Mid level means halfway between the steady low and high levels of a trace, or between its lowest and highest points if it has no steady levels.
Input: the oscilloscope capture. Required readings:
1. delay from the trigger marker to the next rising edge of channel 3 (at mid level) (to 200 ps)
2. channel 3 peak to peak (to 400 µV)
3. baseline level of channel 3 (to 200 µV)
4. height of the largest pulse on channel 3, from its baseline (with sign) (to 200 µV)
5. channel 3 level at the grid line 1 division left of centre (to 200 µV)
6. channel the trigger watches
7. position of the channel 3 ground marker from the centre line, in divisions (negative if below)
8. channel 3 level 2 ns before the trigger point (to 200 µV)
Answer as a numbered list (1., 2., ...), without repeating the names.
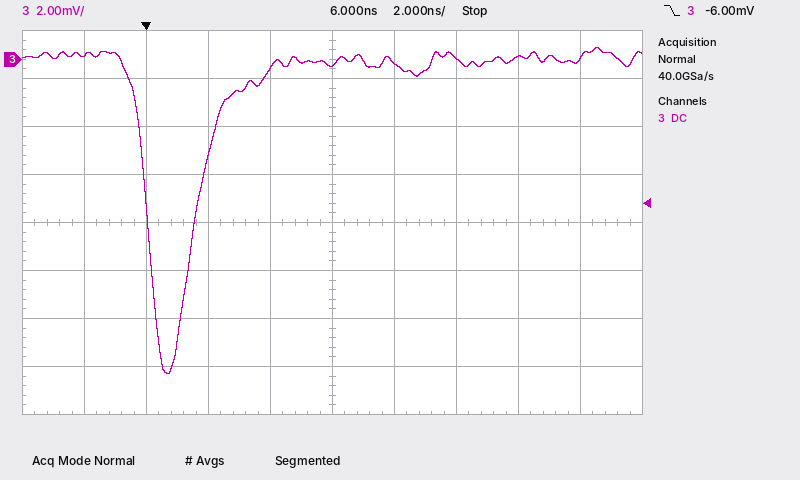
1. 1.6 ns
2. 13.6 mV
3. 0.0 mV
4. -13.0 mV
5. -400 µV
6. channel 3
7. +3.4 div
8. 200 µV
